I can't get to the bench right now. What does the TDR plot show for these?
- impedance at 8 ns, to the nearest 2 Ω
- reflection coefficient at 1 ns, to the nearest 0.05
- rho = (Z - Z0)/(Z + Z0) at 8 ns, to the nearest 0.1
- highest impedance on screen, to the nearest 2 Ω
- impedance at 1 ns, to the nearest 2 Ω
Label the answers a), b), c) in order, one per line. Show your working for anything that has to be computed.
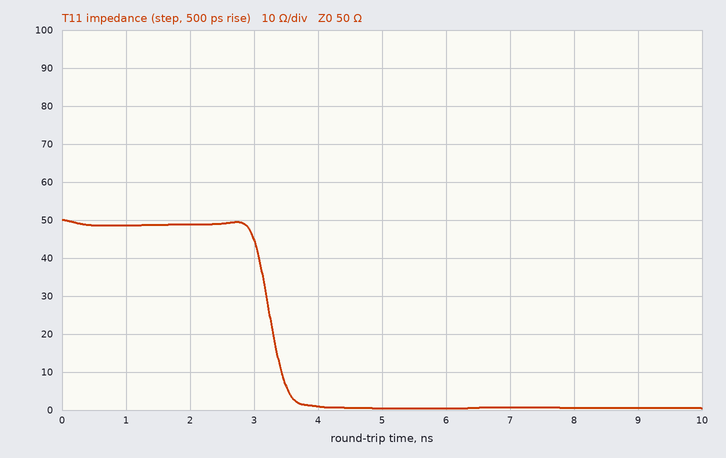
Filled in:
a) 0 Ω
b) (48 − 50)/(48 + 50) ≈ 0.00
c) (0 − 50)/(0 + 50) ≈ -1.0
d) 50 Ω
e) 48 Ω
